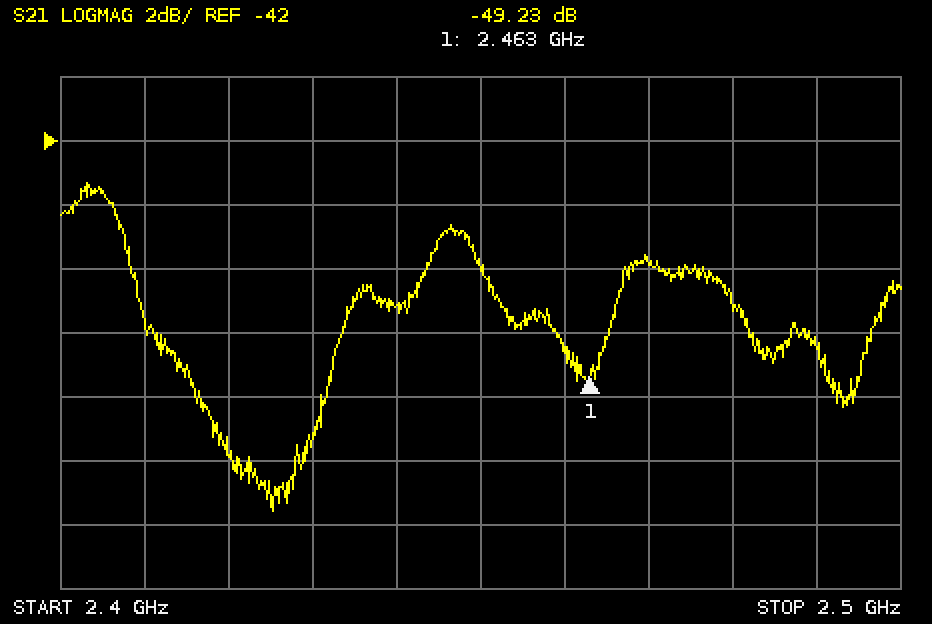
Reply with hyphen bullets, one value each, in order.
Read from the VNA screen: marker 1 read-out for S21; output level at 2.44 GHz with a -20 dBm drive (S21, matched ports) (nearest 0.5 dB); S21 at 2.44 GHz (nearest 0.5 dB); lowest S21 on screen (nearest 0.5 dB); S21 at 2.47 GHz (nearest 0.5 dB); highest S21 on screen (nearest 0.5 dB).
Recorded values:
- -49.23 dB
- -67.0 dBm
- -47.0 dB
- -53.5 dB
- -46.0 dB
- -43.5 dB
